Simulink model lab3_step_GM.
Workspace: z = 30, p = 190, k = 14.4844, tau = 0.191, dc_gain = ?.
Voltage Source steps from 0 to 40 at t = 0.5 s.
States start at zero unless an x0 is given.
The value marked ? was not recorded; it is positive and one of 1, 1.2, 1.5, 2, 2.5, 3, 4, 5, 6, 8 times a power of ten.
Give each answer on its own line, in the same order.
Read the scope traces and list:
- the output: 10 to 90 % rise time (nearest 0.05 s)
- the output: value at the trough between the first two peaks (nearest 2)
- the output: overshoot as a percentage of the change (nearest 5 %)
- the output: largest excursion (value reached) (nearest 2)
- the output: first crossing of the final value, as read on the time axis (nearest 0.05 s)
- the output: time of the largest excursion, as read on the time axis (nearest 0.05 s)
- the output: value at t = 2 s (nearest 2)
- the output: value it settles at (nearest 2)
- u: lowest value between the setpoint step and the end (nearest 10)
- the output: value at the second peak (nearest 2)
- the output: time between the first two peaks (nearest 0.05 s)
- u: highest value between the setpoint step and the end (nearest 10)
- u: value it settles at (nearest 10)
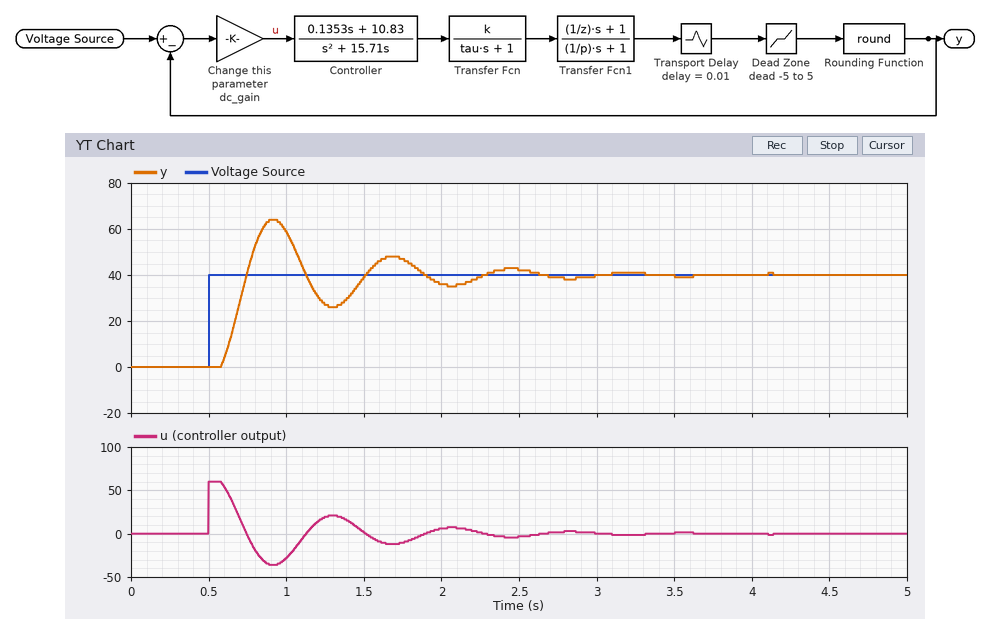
0.15 s
26
60 %
64
0.75 s
0.90 s
36
40
-40
48
0.75 s
60
0
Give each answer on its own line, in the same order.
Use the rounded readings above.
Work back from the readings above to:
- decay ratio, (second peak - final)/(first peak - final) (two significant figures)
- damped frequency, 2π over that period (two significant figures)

0.33
8.4 rad/s
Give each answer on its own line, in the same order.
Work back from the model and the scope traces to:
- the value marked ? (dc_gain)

1.5
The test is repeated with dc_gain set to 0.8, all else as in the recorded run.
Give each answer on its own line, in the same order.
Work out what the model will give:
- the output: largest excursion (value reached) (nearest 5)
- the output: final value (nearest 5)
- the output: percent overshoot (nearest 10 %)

55
40
40 %
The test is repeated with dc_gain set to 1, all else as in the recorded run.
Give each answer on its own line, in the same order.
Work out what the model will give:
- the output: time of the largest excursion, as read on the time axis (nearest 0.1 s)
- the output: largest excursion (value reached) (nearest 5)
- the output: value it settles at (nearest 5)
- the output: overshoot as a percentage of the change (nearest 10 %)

1.0 s
60
40
50 %
